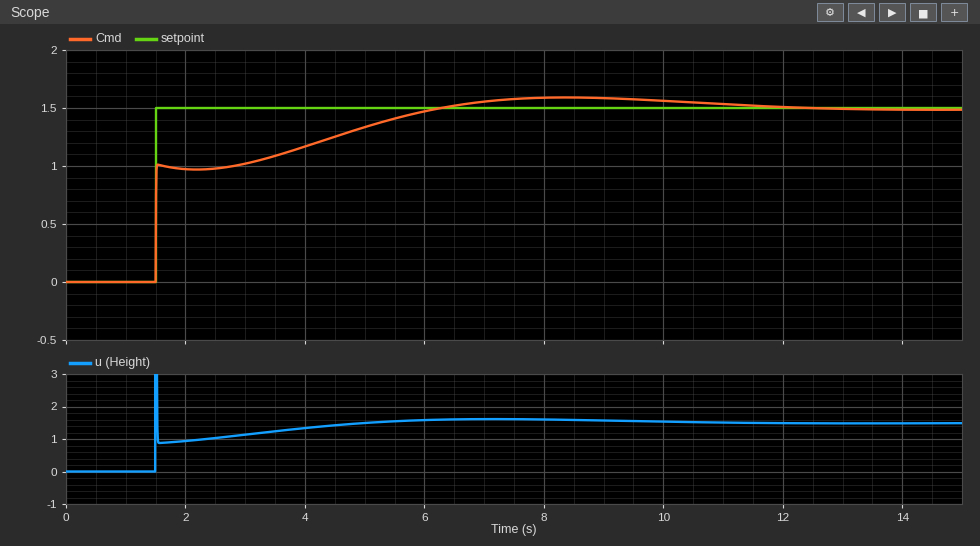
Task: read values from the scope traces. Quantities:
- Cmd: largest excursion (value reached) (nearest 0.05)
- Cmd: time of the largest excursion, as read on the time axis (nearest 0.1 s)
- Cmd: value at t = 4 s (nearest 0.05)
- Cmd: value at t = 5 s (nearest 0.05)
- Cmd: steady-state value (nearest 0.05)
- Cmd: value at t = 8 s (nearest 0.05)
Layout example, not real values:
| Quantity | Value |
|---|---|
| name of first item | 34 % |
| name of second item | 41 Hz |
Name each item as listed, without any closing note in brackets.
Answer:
| Quantity | Value |
|---|---|
| Cmd: largest excursion (value reached) | 1.60 |
| Cmd: time of the largest excursion, as read on the time axis | 8.4 s |
| Cmd: value at t = 4 s | 1.15 |
| Cmd: value at t = 5 s | 1.35 |
| Cmd: steady-state value | 1.50 |
| Cmd: value at t = 8 s | 1.60 |
